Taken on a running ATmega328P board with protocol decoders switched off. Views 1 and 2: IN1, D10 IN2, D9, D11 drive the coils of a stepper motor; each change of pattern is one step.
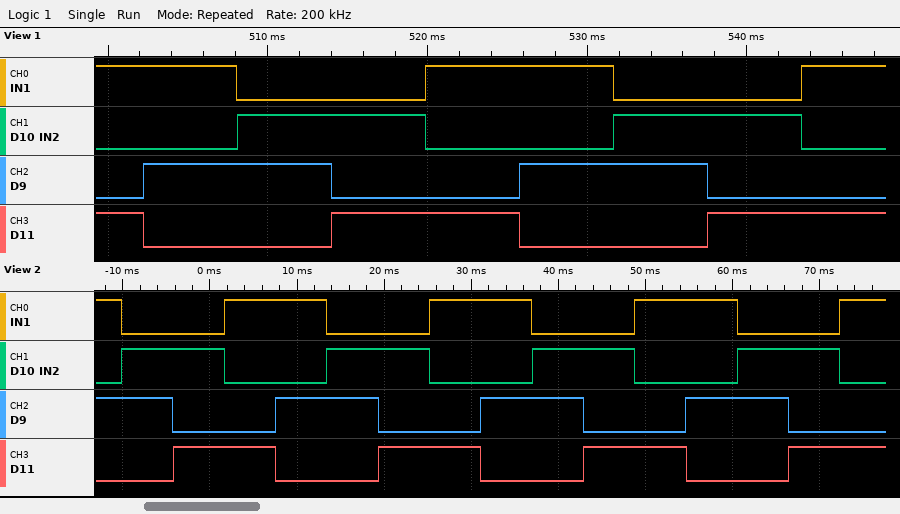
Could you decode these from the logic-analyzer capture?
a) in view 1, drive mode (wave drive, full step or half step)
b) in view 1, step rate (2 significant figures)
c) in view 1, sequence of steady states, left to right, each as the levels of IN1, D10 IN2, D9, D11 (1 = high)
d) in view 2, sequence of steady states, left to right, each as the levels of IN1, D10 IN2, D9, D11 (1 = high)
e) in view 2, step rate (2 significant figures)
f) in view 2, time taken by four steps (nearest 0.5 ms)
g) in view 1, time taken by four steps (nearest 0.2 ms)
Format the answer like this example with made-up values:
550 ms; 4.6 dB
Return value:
full step; 170 steps/s; 1001 1010 0110 0101 1001 1010 0110 0101 1001; 1010 0110 0101 1001 1010 0110 0101 1001 1010 0110 0101 1001 1010 0110 0101 1001; 170 steps/s; 23.5 ms; 23.6 ms
